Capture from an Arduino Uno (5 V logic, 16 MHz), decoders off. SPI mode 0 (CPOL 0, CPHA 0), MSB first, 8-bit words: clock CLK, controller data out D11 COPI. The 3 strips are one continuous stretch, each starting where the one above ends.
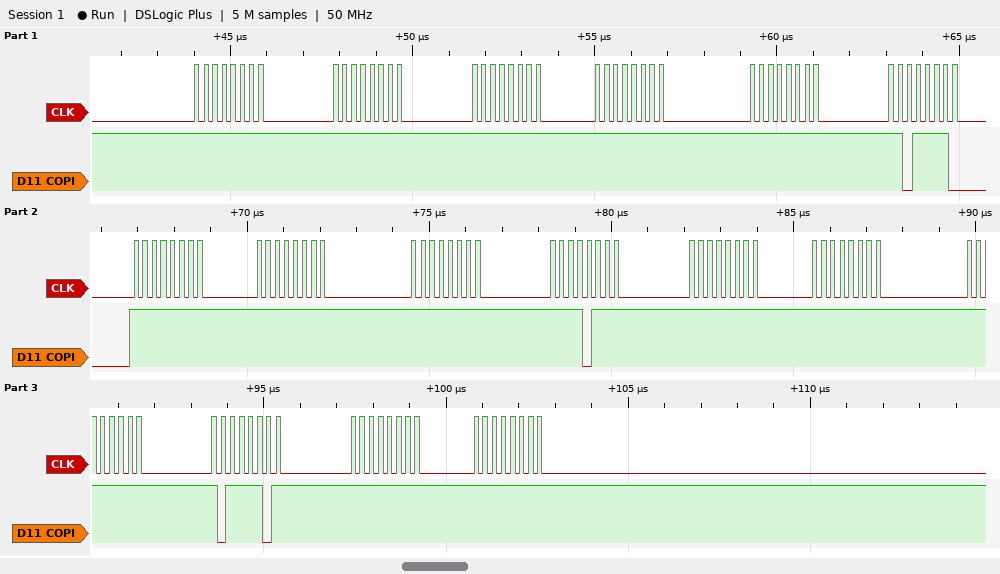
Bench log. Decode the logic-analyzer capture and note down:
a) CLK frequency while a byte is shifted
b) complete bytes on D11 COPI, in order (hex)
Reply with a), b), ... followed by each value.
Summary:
a) 4 MHz
b) 0xFF 0xFF 0xFF 0xFF 0xFF 0xDE 0xFF 0xFF 0xFF 0xF7 0xFF 0xFF 0xFF 0xBD 0xFF 0xFF
